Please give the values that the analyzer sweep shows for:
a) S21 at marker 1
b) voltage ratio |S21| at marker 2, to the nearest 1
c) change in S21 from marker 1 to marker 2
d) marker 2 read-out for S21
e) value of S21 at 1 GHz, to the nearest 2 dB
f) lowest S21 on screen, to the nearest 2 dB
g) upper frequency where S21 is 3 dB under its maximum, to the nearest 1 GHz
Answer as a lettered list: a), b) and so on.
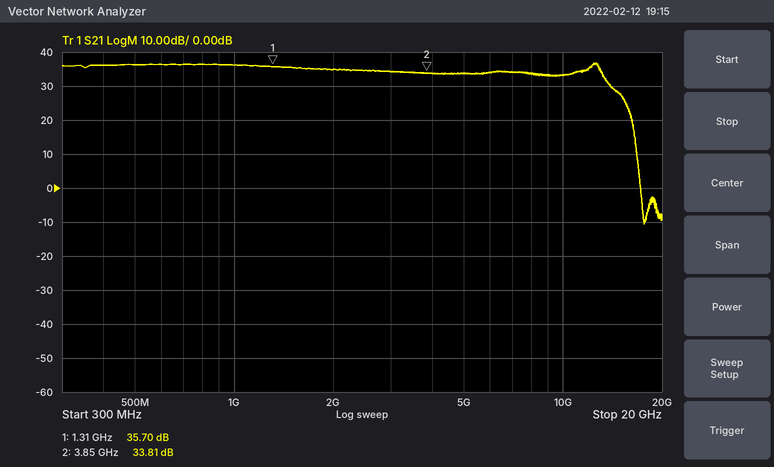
a) 35.70 dB
b) 49
c) -1.89 dB
d) 33.81 dB
e) 36 dB
f) -10 dB
g) 13 GHz
